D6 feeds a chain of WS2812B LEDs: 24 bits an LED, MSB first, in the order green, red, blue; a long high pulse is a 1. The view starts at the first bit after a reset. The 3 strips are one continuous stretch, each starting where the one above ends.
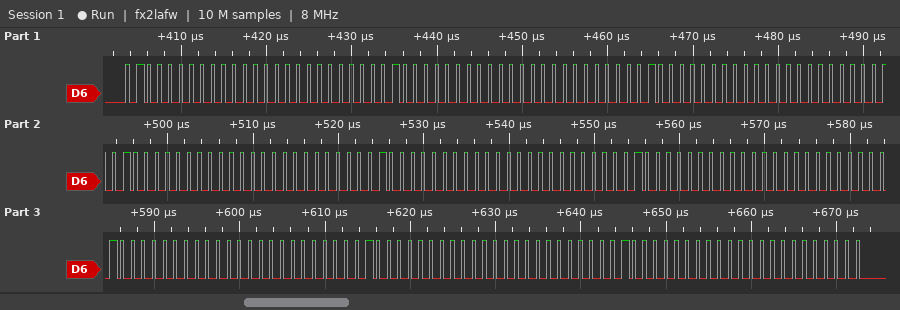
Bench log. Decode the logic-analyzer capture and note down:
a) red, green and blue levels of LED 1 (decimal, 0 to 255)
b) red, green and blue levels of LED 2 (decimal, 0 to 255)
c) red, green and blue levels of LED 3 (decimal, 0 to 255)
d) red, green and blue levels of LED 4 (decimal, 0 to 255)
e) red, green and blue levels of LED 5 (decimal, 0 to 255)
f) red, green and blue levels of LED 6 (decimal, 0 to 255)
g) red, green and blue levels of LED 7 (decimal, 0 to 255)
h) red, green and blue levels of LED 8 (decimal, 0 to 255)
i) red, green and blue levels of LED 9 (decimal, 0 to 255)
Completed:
0, 64, 0
0, 64, 0
0, 64, 0
0, 64, 0
0, 64, 0
0, 64, 0
0, 64, 0
0, 64, 0
0, 64, 0
